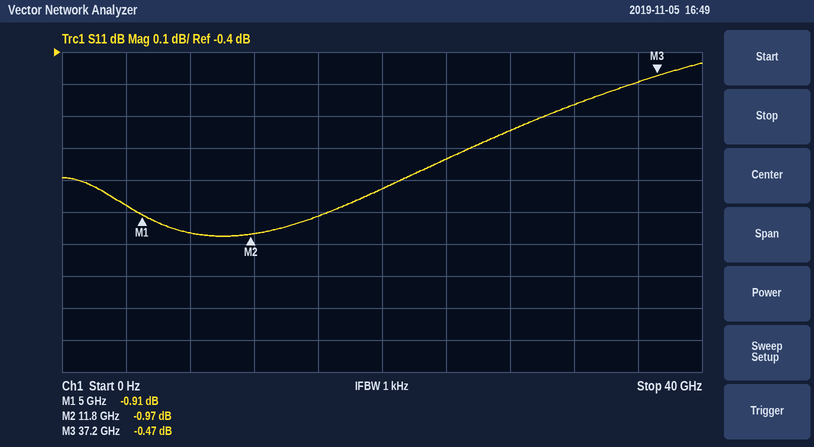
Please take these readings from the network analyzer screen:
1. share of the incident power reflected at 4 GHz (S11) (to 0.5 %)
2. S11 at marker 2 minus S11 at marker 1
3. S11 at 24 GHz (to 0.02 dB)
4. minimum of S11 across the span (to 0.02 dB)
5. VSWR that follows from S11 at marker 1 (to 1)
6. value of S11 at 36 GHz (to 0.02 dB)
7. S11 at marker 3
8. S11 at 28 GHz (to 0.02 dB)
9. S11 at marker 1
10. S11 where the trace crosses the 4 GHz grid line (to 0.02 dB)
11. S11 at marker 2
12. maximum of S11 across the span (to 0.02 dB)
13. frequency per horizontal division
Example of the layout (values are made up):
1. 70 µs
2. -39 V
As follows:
1. 81.5 %
2. -0.06 dB
3. -0.74 dB
4. -0.98 dB
5. 19
6. -0.50 dB
7. -0.47 dB
8. -0.64 dB
9. -0.91 dB
10. -0.88 dB
11. -0.97 dB
12. -0.44 dB
13. 4 GHz
